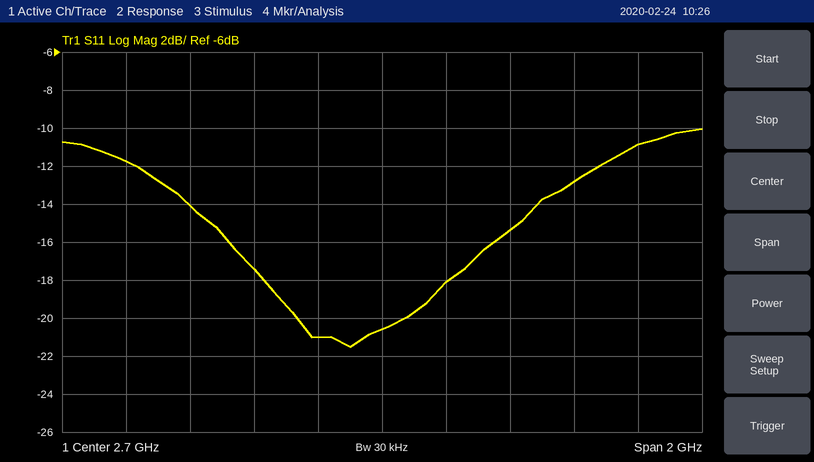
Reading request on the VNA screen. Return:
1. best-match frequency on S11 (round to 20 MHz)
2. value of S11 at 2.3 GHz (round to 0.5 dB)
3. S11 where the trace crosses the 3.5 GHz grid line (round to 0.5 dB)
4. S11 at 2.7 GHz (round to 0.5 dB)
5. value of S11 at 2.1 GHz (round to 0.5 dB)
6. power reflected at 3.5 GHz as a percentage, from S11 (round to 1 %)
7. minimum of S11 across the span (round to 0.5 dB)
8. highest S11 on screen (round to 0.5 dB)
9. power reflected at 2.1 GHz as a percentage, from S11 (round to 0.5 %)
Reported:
2.60 GHz
-17.5 dB
-11.0 dB
-20.5 dB
-14.0 dB
8 %
-21.5 dB
-10.0 dB
4.0 %
